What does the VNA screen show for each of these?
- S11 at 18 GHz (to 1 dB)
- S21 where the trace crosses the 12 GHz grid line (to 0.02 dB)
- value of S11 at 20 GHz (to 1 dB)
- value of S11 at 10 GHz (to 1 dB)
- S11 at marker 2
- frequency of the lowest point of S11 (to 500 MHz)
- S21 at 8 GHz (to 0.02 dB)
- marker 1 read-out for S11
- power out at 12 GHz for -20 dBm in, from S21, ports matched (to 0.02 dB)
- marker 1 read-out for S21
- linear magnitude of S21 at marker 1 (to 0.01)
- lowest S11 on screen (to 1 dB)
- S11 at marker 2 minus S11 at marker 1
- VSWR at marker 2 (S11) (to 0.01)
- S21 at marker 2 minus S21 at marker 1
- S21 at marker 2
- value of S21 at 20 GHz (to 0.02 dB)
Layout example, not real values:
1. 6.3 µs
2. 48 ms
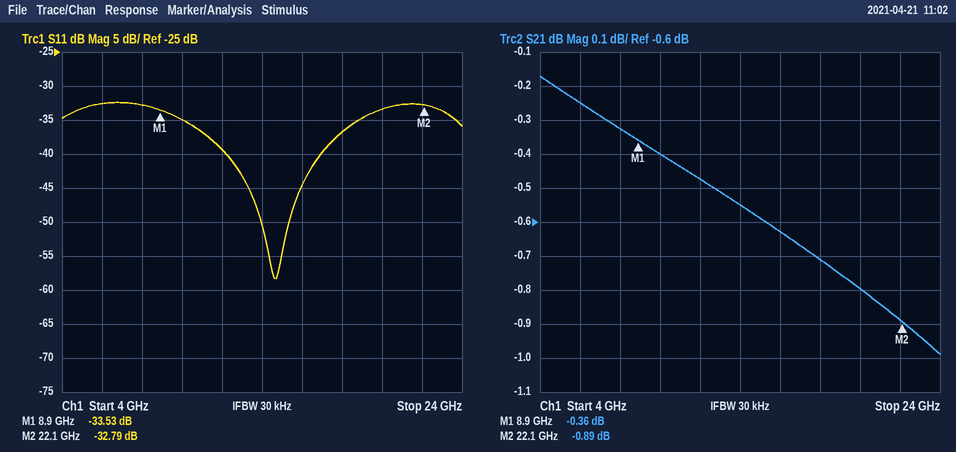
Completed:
1. -37 dB
2. -0.48 dB
3. -33 dB
4. -35 dB
5. -32.79 dB
6. 14.5 GHz
7. -0.32 dB
8. -33.53 dB
9. -20.48 dBm
10. -0.36 dB
11. 0.96
12. -58 dB
13. 0.74 dB
14. 1.05
15. -0.53 dB
16. -0.89 dB
17. -0.80 dB
